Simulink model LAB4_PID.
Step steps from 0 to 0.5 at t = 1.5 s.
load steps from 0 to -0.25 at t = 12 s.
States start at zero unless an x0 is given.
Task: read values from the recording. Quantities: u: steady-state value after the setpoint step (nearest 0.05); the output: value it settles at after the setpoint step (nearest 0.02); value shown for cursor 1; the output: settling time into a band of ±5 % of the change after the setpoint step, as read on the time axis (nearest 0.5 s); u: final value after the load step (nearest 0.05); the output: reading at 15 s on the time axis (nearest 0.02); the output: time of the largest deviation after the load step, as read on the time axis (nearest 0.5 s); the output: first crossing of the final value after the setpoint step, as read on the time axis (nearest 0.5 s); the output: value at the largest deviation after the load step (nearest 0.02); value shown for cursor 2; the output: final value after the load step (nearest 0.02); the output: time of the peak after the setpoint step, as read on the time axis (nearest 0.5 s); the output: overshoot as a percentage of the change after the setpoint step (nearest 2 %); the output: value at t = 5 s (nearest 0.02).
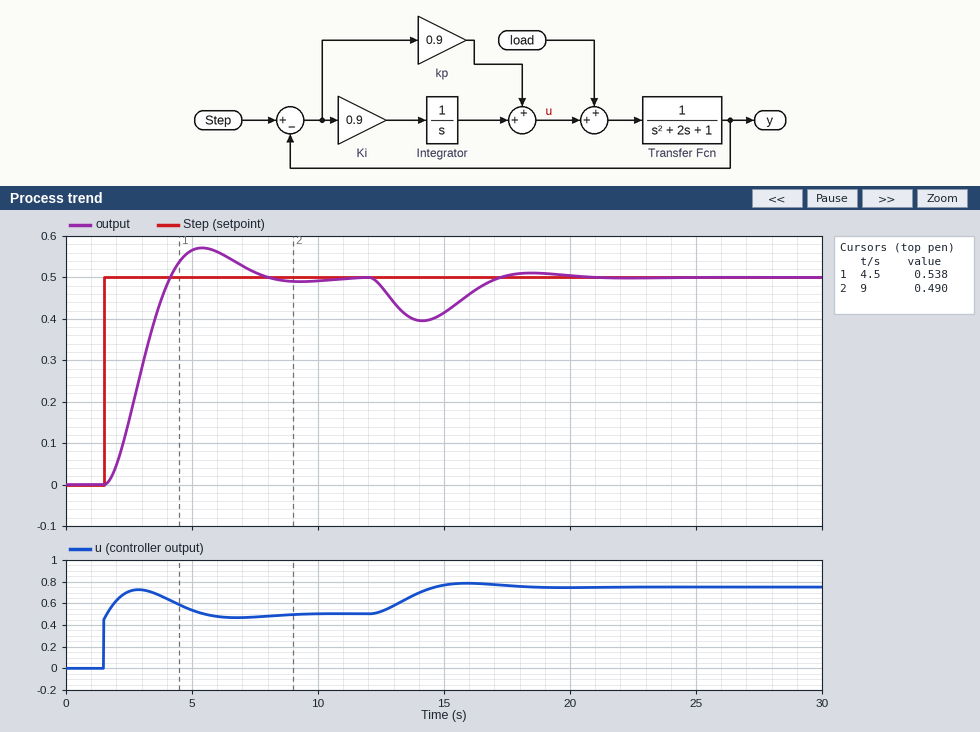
0.50
0.50
0.538
7.0 s
0.75
0.42
14.0 s
4.0 s
0.40
0.490
0.50
5.5 s
14 %
0.56
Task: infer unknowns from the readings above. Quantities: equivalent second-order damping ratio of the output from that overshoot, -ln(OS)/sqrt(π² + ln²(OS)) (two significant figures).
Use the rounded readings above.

0.53
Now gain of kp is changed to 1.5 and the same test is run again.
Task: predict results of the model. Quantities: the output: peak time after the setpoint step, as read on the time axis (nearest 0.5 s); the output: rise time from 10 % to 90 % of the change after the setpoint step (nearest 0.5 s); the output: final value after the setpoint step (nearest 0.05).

4.5 s
1.5 s
0.50
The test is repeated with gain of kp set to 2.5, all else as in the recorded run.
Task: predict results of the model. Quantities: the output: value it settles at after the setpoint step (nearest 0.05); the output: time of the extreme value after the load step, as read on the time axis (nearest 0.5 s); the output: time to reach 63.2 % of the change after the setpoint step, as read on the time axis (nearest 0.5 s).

0.50
13.5 s
2.5 s
